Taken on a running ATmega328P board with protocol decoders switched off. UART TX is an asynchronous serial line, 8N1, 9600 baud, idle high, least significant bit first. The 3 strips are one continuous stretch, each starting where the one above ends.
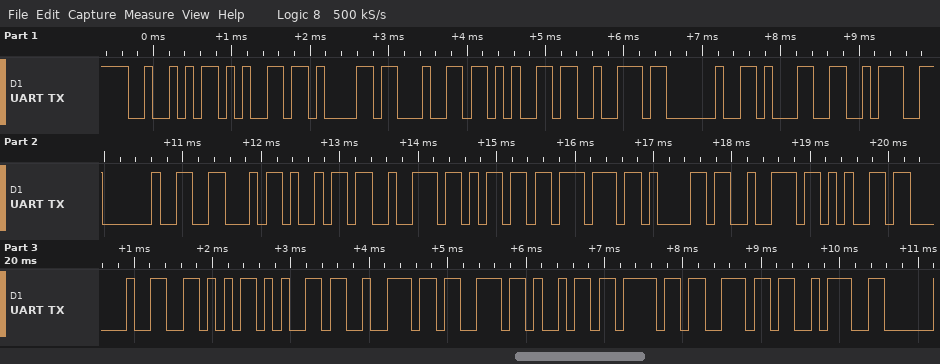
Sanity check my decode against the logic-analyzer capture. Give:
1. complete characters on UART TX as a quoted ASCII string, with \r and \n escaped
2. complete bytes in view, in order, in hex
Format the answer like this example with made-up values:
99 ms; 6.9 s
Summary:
"Reader 1: Firmware Version:"; 0x52 0x65 0x61 0x64 0x65 0x72 0x20 0x31 0x3A 0x20 0x46 0x69 0x72 0x6D 0x77 0x61 0x72 0x65 0x20 0x56 0x65 0x72 0x73 0x69 0x6F 0x6E 0x3A
